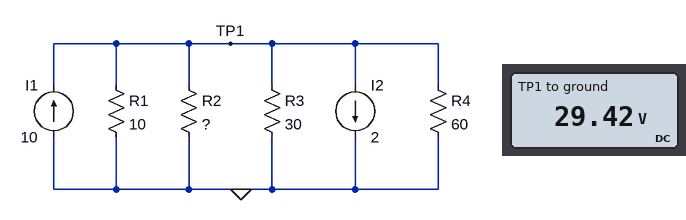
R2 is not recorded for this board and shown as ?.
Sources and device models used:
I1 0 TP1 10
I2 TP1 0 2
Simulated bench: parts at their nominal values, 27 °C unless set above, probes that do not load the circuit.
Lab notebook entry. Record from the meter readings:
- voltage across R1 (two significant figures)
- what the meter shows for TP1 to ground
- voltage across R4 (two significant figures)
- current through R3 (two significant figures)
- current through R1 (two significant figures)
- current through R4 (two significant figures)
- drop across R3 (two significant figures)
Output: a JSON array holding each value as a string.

["29 V", "29.42 V", "29 V", "980 mA", "2.9 A", "490 mA", "29 V"]
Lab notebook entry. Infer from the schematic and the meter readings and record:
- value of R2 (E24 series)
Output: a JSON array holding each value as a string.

["8.2 Ω"]
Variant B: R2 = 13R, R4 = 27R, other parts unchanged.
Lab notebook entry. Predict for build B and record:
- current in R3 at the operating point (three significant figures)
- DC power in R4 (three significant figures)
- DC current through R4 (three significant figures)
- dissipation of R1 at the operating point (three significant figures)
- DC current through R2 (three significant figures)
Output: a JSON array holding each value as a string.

["1.08 A", "38.8 W", "1.20 A", "105 W", "2.49 A"]
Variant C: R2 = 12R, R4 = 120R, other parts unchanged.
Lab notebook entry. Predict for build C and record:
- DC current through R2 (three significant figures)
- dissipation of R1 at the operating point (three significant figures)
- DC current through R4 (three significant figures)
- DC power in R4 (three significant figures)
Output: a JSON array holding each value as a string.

["2.96 A", "126 W", "296 mA", "10.5 W"]
